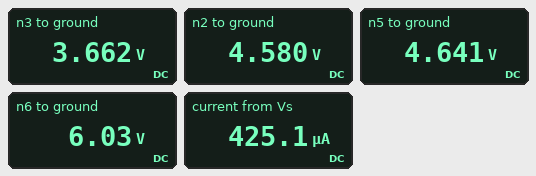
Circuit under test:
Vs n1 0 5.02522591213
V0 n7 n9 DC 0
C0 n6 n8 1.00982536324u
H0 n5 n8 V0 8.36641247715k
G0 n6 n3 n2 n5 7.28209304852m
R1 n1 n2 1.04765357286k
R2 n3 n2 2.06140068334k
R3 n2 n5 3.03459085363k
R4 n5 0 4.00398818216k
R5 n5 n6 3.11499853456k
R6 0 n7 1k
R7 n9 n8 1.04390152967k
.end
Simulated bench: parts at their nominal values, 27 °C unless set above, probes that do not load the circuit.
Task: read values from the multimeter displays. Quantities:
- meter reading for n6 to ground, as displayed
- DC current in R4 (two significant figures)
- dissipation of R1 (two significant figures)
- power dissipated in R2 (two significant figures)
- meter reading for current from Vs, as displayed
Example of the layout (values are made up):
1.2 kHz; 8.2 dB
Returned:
6.03 V; 1.2 mA; 190 µW; 410 µW; 425.1 µA
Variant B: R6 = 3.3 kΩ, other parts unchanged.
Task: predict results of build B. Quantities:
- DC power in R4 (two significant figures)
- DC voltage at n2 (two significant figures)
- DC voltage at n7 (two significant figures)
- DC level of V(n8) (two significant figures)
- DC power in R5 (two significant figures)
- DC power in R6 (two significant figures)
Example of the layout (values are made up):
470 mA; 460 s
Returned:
6.3 mW; 5.0 V; -4.1 V; -5.4 V; 110 nW; 5.1 mW
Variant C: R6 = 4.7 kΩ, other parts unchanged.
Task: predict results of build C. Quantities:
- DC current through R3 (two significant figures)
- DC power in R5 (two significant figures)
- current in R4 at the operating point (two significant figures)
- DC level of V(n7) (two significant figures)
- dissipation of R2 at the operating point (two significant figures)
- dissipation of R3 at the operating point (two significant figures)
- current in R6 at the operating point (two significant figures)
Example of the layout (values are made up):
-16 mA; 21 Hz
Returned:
36 µA; 1.9 mW; 1.4 mA; -10 V; 1.3 mW; 3.8 µW; 2.2 mA
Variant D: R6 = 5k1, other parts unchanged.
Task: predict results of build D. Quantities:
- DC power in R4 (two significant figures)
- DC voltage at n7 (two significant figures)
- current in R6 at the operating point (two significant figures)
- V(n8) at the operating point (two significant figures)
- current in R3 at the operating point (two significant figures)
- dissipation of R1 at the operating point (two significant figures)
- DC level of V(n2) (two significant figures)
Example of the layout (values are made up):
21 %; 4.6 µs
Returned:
9.4 mW; -14 V; 2.8 mA; -17 V; 58 µA; 1.6 mW; 6.3 V
